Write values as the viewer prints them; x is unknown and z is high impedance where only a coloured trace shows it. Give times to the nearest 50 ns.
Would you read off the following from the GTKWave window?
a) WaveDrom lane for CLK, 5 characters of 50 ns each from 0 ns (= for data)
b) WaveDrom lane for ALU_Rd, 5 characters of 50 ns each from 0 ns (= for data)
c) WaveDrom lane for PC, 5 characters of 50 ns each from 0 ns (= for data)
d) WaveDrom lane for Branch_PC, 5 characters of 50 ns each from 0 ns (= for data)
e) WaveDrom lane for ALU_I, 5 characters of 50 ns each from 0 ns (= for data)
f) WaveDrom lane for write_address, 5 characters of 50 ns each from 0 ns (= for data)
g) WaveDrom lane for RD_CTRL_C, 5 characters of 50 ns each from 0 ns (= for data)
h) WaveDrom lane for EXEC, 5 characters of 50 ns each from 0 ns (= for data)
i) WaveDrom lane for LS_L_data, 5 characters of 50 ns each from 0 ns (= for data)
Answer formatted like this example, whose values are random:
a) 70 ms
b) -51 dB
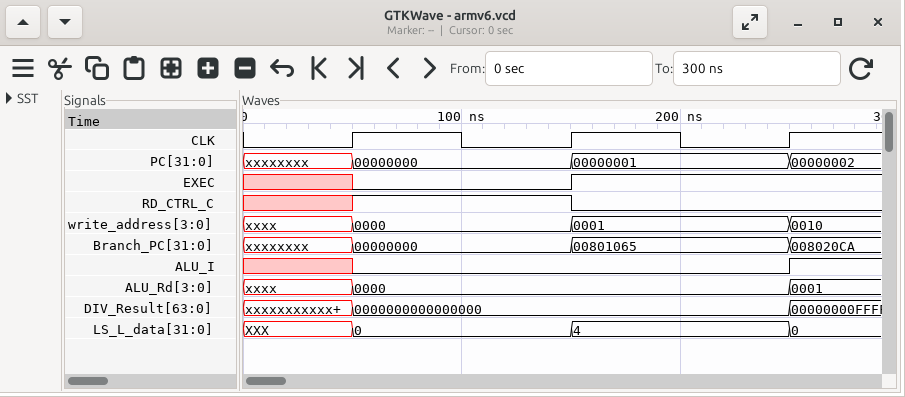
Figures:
a) {name: 'CLK', wave: '01010'}
b) {name: 'ALU_Rd', wave: 'x=...', data: '0000'}
c) {name: 'PC', wave: 'x=.=.', data: '00000000 00000001'}
d) {name: 'Branch_PC', wave: 'x=.=.', data: '00000000 00801065'}
e) {name: 'ALU_I', wave: 'x0...'}
f) {name: 'write_address', wave: 'x=.=.', data: '0000 0001'}
g) {name: 'RD_CTRL_C', wave: 'x1.0.'}
h) {name: 'EXEC', wave: 'x0.1.'}
i) {name: 'LS_L_data', wave: 'x=.=.', data: '0 4'}
